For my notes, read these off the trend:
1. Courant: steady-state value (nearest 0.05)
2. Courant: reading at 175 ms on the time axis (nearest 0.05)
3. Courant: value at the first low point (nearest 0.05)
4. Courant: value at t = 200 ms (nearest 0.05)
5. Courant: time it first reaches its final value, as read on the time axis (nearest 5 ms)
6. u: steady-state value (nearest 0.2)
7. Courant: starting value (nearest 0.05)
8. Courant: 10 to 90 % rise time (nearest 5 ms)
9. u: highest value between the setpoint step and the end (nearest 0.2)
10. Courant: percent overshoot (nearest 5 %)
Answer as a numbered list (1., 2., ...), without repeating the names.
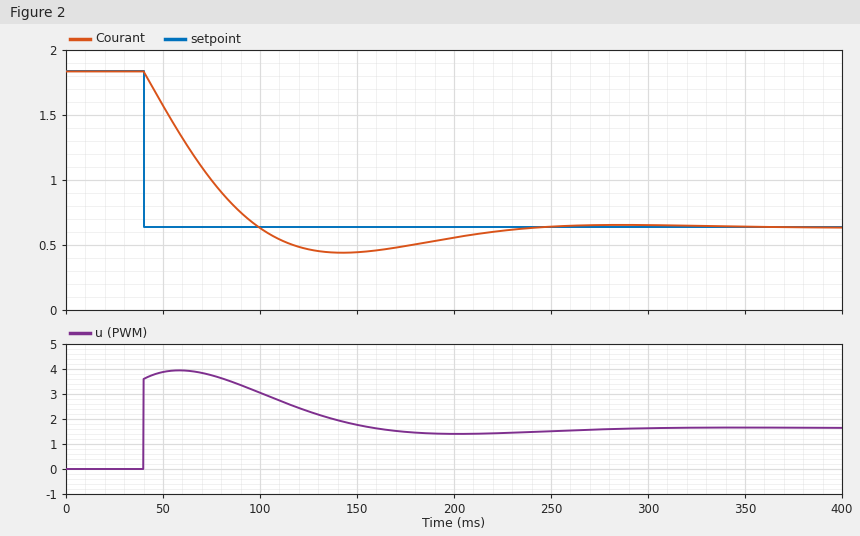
1. 0.65
2. 0.50
3. 0.45
4. 0.55
5. 100 ms
6. 1.6
7. 1.85
8. 45 ms
9. 4.0
10. 15 %
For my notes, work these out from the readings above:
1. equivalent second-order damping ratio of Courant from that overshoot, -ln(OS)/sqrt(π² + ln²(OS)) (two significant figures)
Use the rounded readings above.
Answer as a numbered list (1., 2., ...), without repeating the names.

1. 0.52
